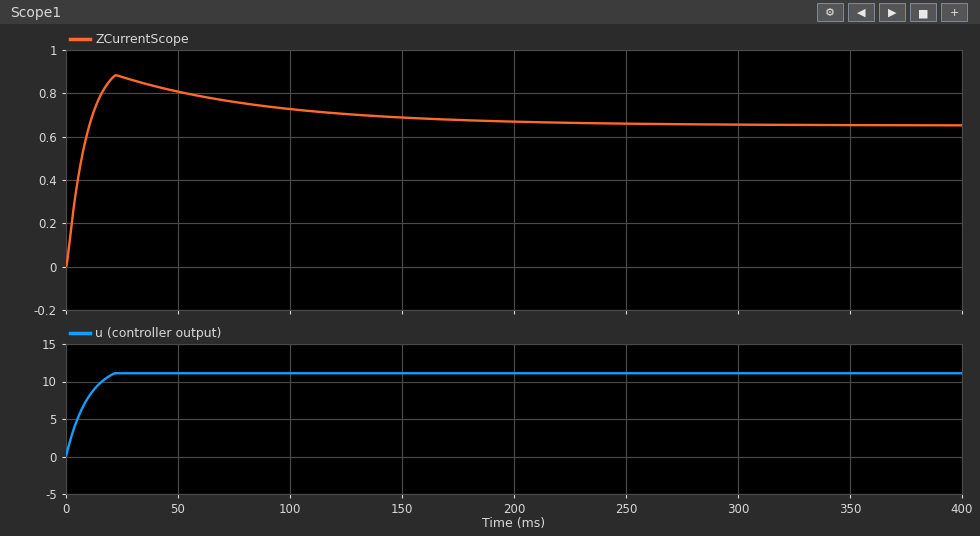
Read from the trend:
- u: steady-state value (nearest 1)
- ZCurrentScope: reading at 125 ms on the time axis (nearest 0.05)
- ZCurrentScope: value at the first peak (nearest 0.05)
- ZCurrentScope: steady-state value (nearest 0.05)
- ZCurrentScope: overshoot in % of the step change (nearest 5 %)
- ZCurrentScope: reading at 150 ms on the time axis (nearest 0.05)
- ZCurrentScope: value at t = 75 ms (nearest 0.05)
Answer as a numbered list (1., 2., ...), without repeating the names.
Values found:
1. 11
2. 0.70
3. 0.90
4. 0.65
5. 35 %
6. 0.70
7. 0.75
